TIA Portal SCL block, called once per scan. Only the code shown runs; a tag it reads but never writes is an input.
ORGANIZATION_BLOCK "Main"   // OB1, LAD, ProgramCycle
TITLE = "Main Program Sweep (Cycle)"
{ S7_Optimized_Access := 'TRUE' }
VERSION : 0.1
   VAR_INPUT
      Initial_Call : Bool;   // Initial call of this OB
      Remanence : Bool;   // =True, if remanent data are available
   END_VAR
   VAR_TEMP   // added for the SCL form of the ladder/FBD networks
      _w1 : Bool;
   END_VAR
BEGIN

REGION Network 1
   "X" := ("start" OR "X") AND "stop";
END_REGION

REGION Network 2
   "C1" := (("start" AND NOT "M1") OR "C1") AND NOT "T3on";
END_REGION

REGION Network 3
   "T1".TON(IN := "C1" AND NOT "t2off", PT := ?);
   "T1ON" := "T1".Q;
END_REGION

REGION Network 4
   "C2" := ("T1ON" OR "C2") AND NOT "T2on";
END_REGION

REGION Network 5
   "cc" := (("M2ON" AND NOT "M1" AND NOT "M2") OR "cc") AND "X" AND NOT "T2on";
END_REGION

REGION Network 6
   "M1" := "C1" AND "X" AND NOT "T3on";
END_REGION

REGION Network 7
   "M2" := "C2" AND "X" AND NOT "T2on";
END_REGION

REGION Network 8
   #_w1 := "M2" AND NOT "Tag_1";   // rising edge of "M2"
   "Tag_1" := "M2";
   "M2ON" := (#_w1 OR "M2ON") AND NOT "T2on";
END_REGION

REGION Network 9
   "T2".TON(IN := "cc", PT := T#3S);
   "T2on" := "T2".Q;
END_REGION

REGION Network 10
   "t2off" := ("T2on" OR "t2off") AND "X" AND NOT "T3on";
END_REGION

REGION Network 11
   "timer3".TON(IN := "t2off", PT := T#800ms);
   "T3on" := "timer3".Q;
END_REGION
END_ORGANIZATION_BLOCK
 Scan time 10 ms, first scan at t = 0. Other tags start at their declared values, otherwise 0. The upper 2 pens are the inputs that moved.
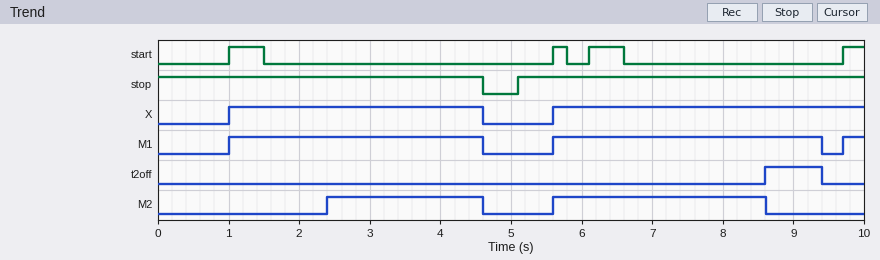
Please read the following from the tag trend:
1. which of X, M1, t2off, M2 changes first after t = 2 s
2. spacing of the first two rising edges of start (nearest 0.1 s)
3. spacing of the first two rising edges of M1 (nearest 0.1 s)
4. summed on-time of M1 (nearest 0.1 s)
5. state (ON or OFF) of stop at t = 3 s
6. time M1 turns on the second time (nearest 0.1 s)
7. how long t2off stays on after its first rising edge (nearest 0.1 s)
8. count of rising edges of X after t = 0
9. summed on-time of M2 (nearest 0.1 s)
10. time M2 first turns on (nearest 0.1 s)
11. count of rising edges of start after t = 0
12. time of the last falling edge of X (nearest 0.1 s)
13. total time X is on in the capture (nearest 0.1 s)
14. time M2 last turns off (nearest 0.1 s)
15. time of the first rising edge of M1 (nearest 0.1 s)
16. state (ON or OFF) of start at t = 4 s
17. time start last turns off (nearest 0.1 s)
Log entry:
M2
4.6 s
4.6 s
7.7 s
ON
5.6 s
0.8 s
2
5.2 s
2.4 s
4
4.6 s
8.0 s
8.6 s
1.0 s
OFF
6.6 s
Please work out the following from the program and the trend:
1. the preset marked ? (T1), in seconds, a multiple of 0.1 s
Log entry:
1.4 s
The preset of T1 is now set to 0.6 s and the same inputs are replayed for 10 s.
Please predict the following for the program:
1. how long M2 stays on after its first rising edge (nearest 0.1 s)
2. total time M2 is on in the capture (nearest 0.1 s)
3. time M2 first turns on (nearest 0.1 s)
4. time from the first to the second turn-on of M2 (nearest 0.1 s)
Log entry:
3.0 s
6.0 s
1.6 s
4.0 s
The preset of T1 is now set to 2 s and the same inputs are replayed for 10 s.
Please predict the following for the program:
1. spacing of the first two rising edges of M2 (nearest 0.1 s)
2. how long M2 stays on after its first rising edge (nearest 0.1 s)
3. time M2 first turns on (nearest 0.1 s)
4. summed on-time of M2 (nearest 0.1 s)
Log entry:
2.6 s
1.6 s
3.0 s
4.6 s
